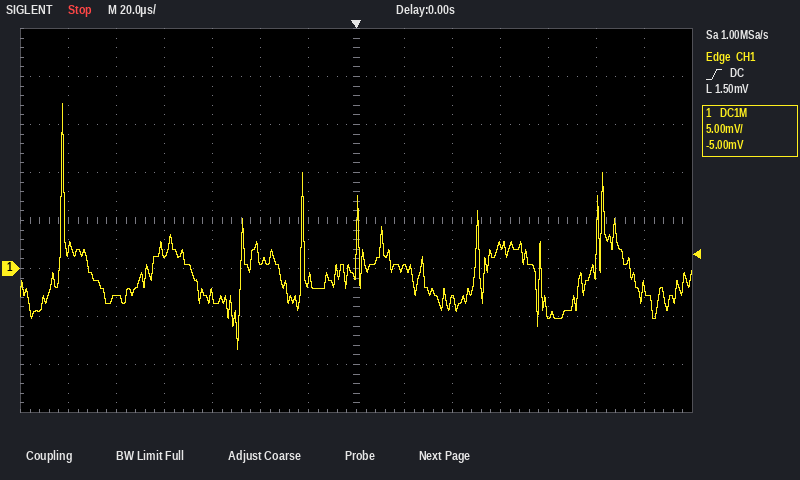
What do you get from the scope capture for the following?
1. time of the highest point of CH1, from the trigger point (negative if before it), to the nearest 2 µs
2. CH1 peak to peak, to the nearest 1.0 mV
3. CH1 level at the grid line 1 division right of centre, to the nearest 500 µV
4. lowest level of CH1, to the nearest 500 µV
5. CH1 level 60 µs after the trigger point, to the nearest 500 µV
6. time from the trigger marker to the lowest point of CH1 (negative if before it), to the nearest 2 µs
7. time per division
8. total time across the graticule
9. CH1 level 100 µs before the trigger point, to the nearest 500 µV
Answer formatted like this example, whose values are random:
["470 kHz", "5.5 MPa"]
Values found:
["-122 µs", "26.0 mV", "0.0 mV", "-8.5 mV", "2.5 mV", "-50 µs", "20 µs", "280 µs", "-3.0 mV"]
